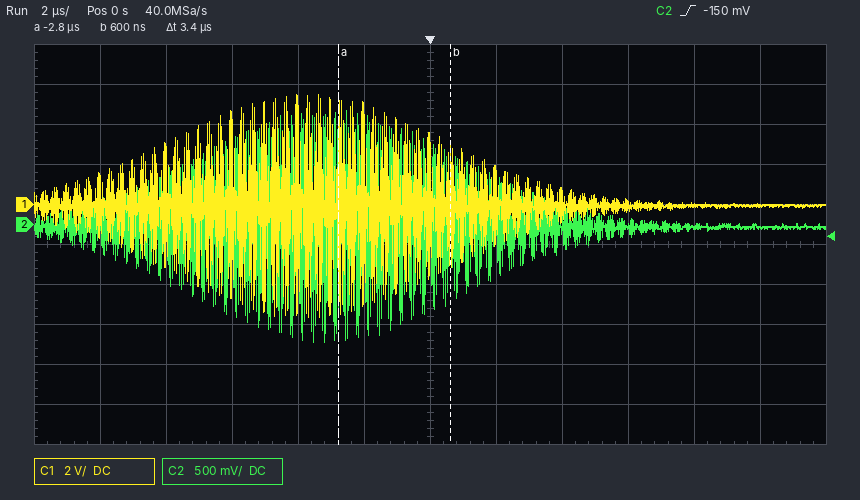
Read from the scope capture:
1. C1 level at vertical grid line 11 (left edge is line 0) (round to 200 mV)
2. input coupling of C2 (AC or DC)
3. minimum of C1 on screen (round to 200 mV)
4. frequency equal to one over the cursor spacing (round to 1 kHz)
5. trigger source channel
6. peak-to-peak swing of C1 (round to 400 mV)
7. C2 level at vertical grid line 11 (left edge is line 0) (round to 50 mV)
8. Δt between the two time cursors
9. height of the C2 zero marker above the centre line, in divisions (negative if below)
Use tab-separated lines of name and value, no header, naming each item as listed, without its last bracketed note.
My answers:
C1 level at vertical grid line 11 (left edge is line 0)	0.0 V
input coupling of C2	DC
minimum of C1 on screen	-5.6 V
frequency equal to one over the cursor spacing	294 kHz
trigger source channel	C2
peak-to-peak swing of C1	11.2 V
C2 level at vertical grid line 11 (left edge is line 0)	-50 mV
Δt between the two time cursors	3.4 µs
height of the C2 zero marker above the centre line, in divisions	+0.5 div
